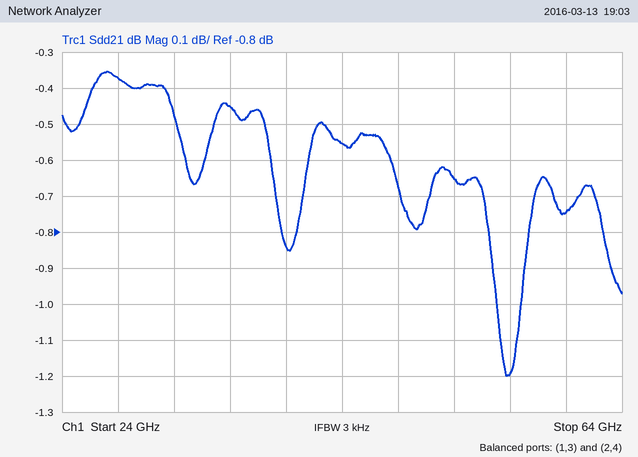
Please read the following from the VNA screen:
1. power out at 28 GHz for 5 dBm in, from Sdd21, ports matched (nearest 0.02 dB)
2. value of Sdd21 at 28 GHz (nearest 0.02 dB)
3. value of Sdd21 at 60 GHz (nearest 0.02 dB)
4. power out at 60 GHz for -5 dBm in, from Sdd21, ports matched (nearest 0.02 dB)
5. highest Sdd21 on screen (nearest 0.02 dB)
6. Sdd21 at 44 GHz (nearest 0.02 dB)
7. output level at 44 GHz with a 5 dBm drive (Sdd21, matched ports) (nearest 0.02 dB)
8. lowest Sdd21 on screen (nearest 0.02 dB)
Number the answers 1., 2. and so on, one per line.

1. 4.62 dBm
2. -0.38 dB
3. -0.74 dB
4. -5.74 dBm
5. -0.36 dB
6. -0.56 dB
7. 4.44 dBm
8. -1.20 dB
